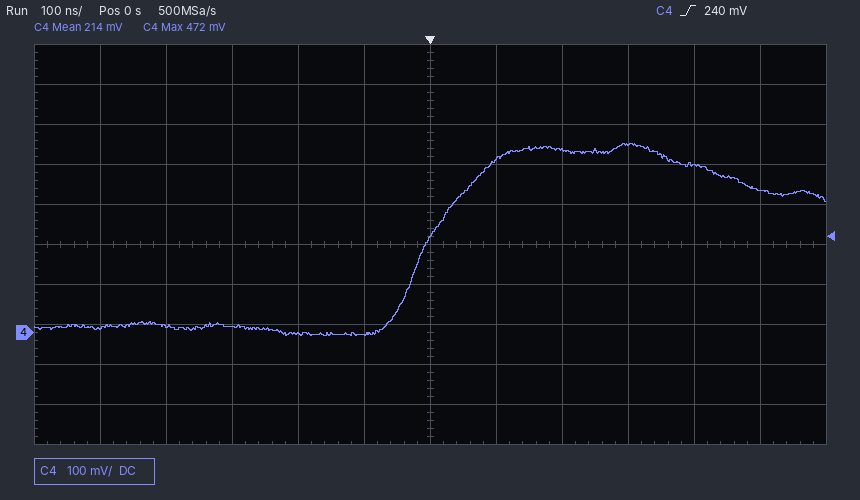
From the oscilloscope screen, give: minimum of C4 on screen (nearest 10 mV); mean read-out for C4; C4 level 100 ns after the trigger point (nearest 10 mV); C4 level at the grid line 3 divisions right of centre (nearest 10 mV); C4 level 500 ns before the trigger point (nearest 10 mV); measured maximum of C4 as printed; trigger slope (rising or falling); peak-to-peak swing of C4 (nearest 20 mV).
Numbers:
-10 mV
214 mV
430 mV
470 mV
10 mV
472 mV
rising
480 mV
